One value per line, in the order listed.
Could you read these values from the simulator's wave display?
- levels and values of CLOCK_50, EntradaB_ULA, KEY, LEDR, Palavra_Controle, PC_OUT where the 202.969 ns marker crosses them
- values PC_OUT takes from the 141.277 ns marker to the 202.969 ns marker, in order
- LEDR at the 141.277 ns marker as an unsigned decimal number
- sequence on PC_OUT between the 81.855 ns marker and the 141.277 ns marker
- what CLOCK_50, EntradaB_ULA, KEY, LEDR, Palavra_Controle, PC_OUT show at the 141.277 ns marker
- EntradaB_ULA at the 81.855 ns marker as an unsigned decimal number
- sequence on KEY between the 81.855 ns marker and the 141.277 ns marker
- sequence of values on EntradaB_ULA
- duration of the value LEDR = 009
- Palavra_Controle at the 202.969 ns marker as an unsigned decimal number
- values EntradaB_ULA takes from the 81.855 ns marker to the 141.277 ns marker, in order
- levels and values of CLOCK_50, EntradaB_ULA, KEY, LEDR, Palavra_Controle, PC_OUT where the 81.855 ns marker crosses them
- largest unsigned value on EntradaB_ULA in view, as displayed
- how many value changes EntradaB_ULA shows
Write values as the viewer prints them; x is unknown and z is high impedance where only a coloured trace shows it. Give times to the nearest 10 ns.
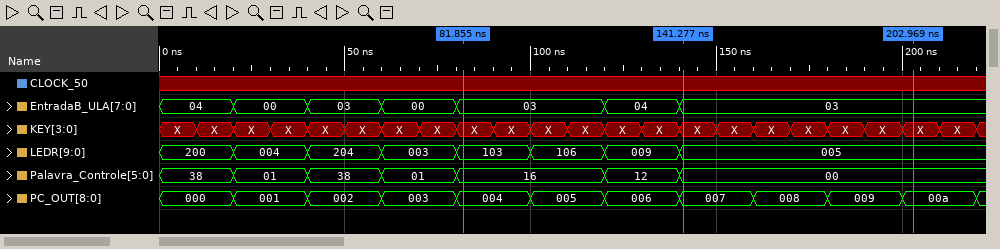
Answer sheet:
CLOCK_50=x, EntradaB_ULA=03, KEY=X, LEDR=005, Palavra_Controle=00, PC_OUT=00a
007, 008, 009, 00a
5
004, 005, 006, 007
CLOCK_50=x, EntradaB_ULA=03, KEY=X, LEDR=005, Palavra_Controle=00, PC_OUT=007
3
X, X, X, X, X, X, X
04, 00, 03, 00, 03, 04, 03
20 ns
0
03, 04, 03
CLOCK_50=x, EntradaB_ULA=03, KEY=X, LEDR=103, Palavra_Controle=16, PC_OUT=004
04
6
